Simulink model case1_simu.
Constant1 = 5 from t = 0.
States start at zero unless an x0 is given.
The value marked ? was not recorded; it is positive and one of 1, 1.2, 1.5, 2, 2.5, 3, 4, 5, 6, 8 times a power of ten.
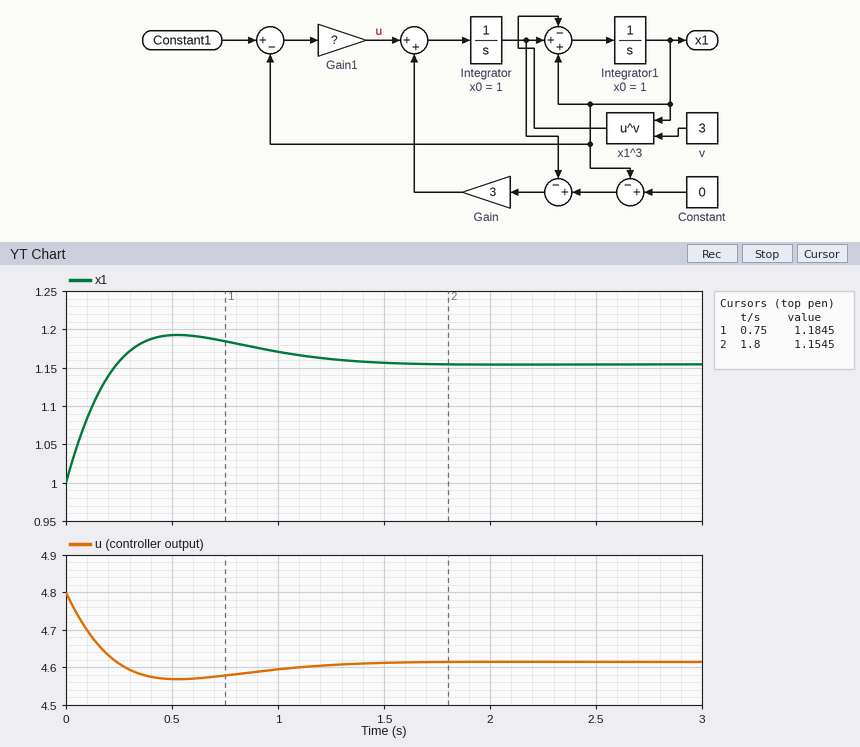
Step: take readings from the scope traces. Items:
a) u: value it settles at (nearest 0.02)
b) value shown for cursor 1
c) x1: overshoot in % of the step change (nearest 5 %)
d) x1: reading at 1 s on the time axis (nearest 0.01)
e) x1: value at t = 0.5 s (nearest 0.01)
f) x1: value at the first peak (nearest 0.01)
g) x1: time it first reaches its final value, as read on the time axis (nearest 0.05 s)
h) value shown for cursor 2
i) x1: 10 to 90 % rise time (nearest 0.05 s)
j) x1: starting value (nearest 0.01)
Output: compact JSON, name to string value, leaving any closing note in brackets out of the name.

{"u: value it settles at": "4.62", "value shown for cursor 1": "1.1845", "x1: overshoot in % of the step change": "25 %", "x1: reading at 1 s on the time axis": "1.17", "x1: value at t = 0.5 s": "1.19", "x1: value at the first peak": "1.19", "x1: time it first reaches its final value, as read on the time axis": "0.25 s", "value shown for cursor 2": "1.1545", "x1: 10 to 90 % rise time": "0.20 s", "x1: starting value": "1.00"}
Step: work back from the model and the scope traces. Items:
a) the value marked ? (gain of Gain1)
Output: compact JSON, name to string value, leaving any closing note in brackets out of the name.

{"the value marked ?": "1.2"}
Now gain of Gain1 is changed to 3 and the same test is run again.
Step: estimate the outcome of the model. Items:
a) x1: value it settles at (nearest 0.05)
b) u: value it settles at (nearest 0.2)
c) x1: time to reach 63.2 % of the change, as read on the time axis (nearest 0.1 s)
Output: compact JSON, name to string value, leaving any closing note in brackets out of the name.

{"x1: value it settles at": "1.50", "u: value it settles at": "10.4", "x1: time to reach 63.2 % of the change, as read on the time axis": "0.3 s"}
